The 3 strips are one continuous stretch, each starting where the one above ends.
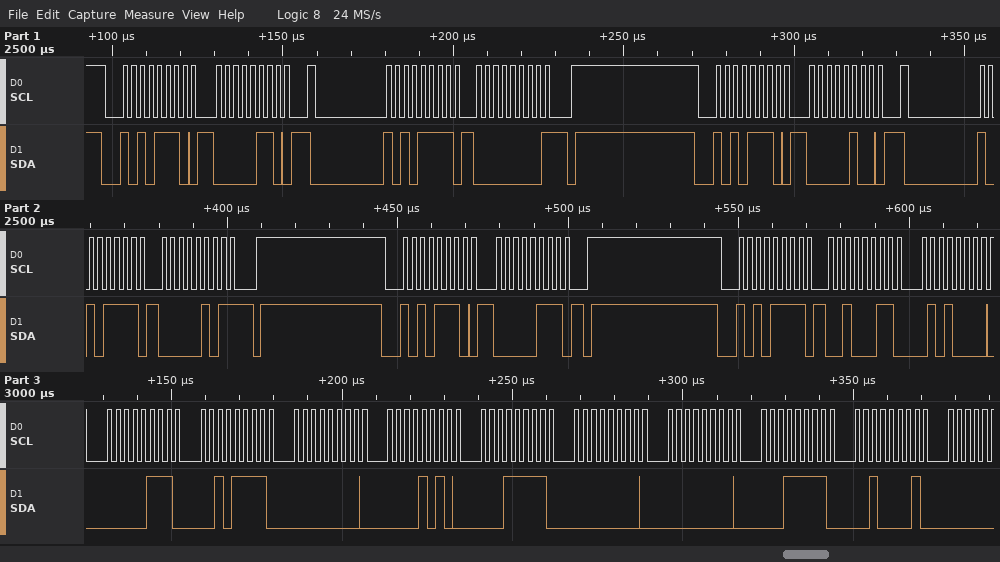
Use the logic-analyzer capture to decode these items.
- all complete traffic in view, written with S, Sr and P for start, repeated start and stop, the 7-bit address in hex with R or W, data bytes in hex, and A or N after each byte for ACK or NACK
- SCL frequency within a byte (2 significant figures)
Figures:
S 57W A 06 A Sr 57R A 00 N P S 57W A 04 A Sr 57R A 05 N P S 57W A 07 A P S 57R A 23 A 50 A 07 A 2F A 00 A 0A A 1F A 00 A 00 A 1F A 21 A
400 kHz
